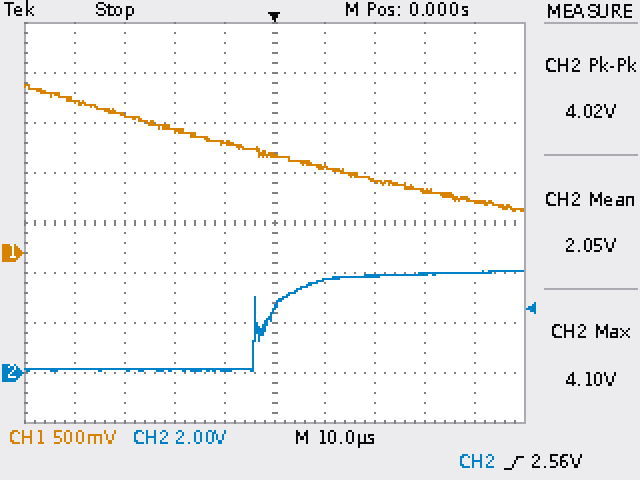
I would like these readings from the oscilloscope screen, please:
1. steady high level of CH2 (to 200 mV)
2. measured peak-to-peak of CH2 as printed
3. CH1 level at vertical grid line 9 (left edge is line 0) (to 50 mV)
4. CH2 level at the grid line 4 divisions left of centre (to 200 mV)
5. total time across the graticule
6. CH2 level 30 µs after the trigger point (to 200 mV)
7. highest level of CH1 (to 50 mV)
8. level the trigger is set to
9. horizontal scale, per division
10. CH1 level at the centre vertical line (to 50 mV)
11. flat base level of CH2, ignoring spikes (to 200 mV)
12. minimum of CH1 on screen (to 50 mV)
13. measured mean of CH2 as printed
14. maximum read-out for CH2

4.0 V
4.02 V
500 mV
200 mV
100 µs
4.0 V
1.70 V
2.56 V
10 µs
1.00 V
200 mV
400 mV
2.05 V
4.10 V
